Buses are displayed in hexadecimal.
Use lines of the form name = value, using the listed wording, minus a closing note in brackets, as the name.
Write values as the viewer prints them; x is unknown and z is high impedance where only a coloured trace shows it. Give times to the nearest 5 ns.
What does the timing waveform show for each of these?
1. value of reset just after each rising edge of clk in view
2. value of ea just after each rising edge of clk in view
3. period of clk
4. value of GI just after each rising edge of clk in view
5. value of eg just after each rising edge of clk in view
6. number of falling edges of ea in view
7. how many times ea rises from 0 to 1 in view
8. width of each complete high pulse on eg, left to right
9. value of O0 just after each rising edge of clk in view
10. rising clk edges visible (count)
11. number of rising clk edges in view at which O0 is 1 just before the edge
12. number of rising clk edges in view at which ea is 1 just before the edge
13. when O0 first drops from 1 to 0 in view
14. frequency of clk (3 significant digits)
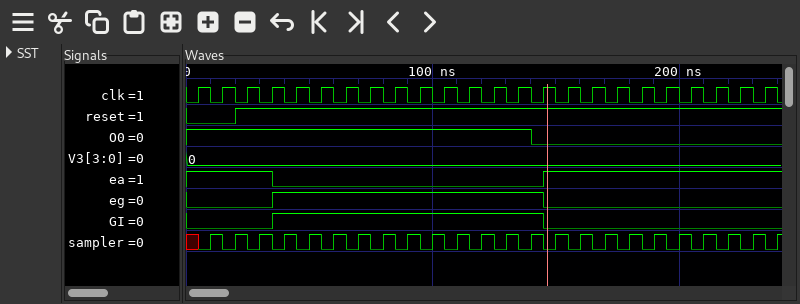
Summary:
value of reset just after each rising edge of clk in view = 0 0 1 1 1 1 1 1 1 1 1 1 1 1 1 1 1 1 1 1 1 1 1 1
value of ea just after each rising edge of clk in view = 1 1 1 0 0 0 0 0 0 0 0 0 0 0 1 1 1 1 1 1 1 1 1 1
period of clk = 10 ns
value of GI just after each rising edge of clk in view = 0 0 0 1 1 1 1 1 1 1 1 1 1 1 0 0 0 0 0 0 0 0 0 0
value of eg just after each rising edge of clk in view = 0 0 0 1 1 1 1 1 1 1 1 1 1 1 0 0 0 0 0 0 0 0 0 0
number of falling edges of ea in view = 1
how many times ea rises from 0 to 1 in view = 1
width of each complete high pulse on eg, left to right = 110 ns
value of O0 just after each rising edge of clk in view = 1 1 1 1 1 1 1 1 1 1 1 1 1 1 0 0 0 0 0 0 0 0 0 0
rising clk edges visible = 24
number of rising clk edges in view at which O0 is 1 just before the edge = 14
number of rising clk edges in view at which ea is 1 just before the edge = 13
when O0 first drops from 1 to 0 in view = 140 ns
frequency of clk = 100 MHz
